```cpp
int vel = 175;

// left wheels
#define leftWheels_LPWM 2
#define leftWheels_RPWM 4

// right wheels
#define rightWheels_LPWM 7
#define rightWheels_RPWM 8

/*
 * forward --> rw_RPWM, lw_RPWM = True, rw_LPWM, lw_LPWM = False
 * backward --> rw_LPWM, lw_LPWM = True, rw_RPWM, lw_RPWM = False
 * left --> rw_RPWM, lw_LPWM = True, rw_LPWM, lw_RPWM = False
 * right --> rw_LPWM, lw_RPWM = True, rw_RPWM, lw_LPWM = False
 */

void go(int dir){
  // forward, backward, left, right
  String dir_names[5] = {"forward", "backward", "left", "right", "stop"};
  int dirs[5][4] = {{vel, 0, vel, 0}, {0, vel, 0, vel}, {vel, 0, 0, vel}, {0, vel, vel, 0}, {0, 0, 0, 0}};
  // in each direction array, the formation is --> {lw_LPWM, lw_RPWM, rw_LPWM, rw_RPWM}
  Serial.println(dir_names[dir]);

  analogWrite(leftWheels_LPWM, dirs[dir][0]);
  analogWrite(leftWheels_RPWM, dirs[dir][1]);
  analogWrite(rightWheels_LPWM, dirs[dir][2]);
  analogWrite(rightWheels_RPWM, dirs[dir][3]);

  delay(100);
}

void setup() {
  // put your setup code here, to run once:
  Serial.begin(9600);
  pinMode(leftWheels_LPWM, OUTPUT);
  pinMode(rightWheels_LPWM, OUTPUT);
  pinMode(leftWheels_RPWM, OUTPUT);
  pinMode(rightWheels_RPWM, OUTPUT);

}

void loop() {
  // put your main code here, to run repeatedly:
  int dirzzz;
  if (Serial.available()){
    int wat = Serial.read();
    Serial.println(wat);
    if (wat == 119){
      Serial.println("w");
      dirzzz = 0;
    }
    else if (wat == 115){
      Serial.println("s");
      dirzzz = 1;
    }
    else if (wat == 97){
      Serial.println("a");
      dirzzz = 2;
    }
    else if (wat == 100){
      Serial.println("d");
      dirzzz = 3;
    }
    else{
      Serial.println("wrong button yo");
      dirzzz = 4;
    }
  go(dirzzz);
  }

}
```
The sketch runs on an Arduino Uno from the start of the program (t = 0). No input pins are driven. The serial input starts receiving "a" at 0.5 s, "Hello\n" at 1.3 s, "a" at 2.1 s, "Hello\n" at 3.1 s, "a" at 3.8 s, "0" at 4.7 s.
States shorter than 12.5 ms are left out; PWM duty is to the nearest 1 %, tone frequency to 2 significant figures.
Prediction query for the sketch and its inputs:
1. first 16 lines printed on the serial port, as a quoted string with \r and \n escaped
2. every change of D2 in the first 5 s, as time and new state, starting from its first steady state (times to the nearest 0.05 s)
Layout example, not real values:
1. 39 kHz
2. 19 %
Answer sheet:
1. "97\r\na\r\nleft\r\n72\r\nwrong button yo\r\nstop\r\n101\r\nwrong button yo\r\nstop\r\n108\r\nwrong button yo\r\nstop\r\n108\r\nwrong button yo\r\nstop\r\n111\r\n"
2. 0 s low; 0.5 s high; 1.3 s low; 2.1 s high; 3.1 s low; 3.8 s high; 4.7 s low
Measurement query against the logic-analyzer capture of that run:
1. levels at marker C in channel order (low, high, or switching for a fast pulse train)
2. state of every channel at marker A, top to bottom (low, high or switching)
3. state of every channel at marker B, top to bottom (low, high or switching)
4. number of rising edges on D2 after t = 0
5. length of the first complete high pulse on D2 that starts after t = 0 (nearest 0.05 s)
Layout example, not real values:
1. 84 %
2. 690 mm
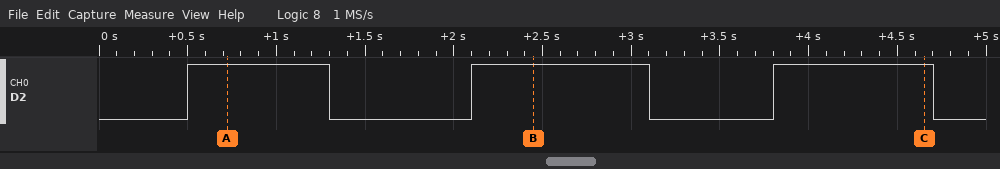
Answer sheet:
1. D2 high
2. D2 high
3. D2 high
4. 3
5. 0.80 s
